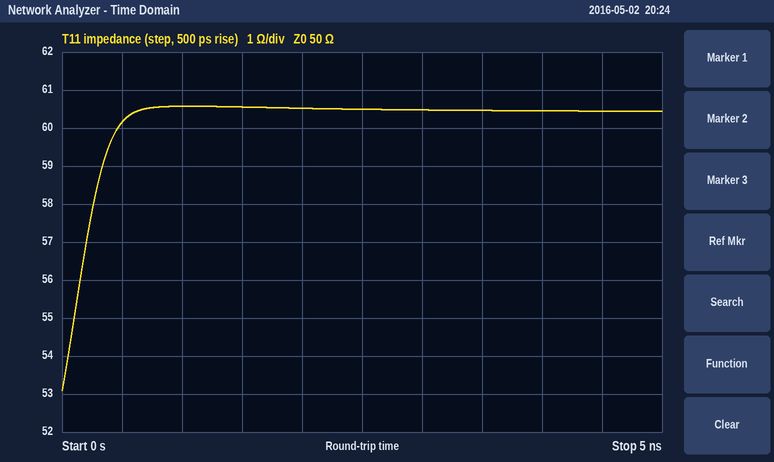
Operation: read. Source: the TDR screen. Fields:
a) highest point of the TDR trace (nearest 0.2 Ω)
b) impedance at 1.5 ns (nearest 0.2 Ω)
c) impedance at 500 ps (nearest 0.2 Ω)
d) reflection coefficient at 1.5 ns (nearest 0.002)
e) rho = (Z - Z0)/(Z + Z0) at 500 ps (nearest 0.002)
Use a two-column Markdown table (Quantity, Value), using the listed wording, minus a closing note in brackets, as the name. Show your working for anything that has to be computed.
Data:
| Quantity | Value |
|---|---|
| highest point of the TDR trace | 60.6 Ω |
| impedance at 1.5 ns | 60.6 Ω |
| impedance at 500 ps | 60.2 Ω |
| reflection coefficient at 1.5 ns | (60.6 − 50)/(60.6 + 50) ≈ +0.096 |
| rho = (Z - Z0)/(Z + Z0) at 500 ps | (60.2 − 50)/(60.2 + 50) ≈ +0.0926, so +0.092 to the nearest 0.002 |
